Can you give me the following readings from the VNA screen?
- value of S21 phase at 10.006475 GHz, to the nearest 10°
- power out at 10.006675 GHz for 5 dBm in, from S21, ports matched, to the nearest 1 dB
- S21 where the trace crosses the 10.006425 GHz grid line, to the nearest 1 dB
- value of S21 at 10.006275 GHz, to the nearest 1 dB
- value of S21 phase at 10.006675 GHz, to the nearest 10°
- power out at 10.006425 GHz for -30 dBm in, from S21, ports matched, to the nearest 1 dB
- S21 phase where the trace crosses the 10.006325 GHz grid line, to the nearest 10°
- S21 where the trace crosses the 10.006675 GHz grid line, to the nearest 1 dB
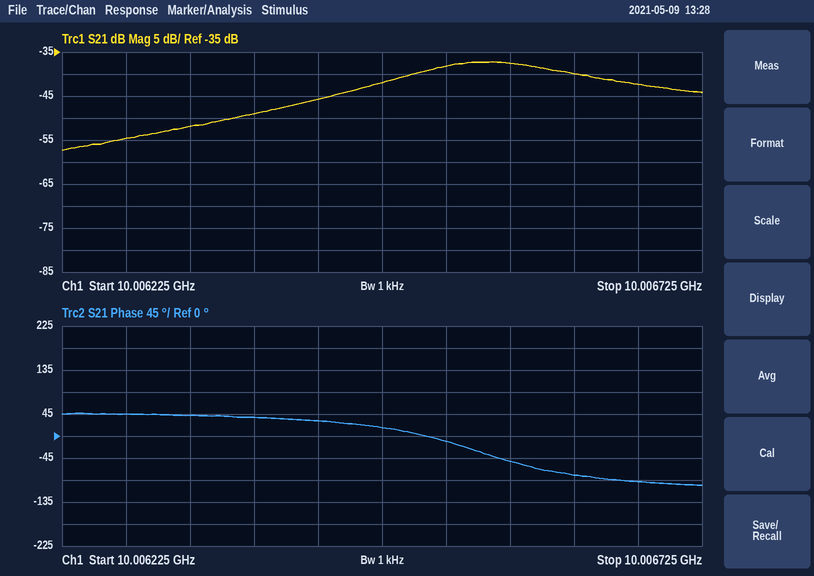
20°
-37 dBm
-46 dB
-55 dB
-90°
-76 dBm
40°
-42 dB
